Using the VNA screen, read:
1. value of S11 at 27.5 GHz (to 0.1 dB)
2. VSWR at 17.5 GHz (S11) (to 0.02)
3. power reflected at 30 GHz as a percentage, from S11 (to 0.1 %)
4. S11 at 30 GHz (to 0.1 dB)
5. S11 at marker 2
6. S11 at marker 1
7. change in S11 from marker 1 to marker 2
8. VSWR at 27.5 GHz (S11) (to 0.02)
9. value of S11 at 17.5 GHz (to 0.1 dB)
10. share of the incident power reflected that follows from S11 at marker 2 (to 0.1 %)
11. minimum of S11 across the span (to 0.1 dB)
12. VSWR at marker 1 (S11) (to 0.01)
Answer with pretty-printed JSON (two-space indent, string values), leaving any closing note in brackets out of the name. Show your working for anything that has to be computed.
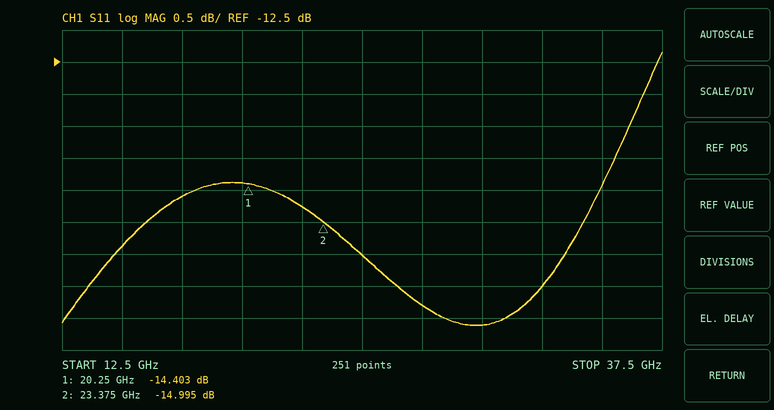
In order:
{
  "value of S11 at 27.5 GHz": "-16.3 dB",
  "VSWR at 17.5 GHz (S11)": "|Γ| = 10^(-14.6/20) = 0.1862; VSWR = (1 + 0.1862)/(1 − 0.1862) ≈ 1.46",
  "power reflected at 30 GHz as a percentage, from S11": "10^(-16.6/10) ≈ 2.2 %",
  "S11 at 30 GHz": "-16.6 dB",
  "S11 at marker 2": "-14.995 dB",
  "S11 at marker 1": "-14.403 dB",
  "change in S11 from marker 1 to marker 2": "-14.995 − (-14.403) = -0.592 dB",
  "VSWR at 27.5 GHz (S11)": "|Γ| = 10^(-16.3/20) = 0.1531; VSWR = (1 + 0.1531)/(1 − 0.1531) ≈ 1.36",
  "value of S11 at 17.5 GHz": "-14.6 dB",
  "share of the incident power reflected that follows from S11 at marker 2": "10^(-14.995/10) ≈ 3.2 %",
  "minimum of S11 across the span": "-16.6 dB",
  "VSWR at marker 1 (S11)": "(1 + 0.1905)/(1 − 0.1905) ≈ 1.47"
}
